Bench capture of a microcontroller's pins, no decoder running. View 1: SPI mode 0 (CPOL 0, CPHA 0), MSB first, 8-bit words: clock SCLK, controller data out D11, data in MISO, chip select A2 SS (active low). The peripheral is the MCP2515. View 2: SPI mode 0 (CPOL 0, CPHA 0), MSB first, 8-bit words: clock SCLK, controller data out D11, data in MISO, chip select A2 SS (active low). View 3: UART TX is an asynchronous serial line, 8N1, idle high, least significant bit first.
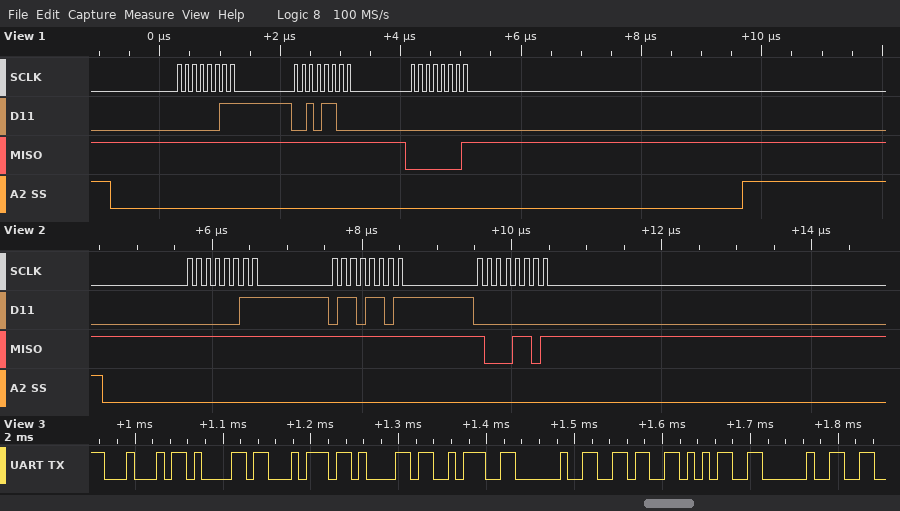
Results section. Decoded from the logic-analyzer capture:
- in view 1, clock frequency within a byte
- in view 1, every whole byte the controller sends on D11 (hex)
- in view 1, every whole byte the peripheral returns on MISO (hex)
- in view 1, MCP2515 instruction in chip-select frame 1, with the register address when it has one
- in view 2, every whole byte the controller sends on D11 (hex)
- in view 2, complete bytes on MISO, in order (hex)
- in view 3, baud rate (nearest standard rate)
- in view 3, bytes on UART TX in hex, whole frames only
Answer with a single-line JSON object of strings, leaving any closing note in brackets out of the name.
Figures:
{"in view 1, clock frequency within a byte": "8 MHz", "in view 1, every whole byte the controller sends on D11": "0x03 0x2C 0x00", "in view 1, every whole byte the peripheral returns on MISO": "0xFF 0xFF 0x01", "in view 1, MCP2515 instruction in chip-select frame 1, with the register address when it has one": "READ 0x2C", "in view 2, every whole byte the controller sends on D11": "03 6D 00", "in view 2, complete bytes on MISO, in order": "FF FF 8D", "in view 3, baud rate": "115200 baud", "in view 3, bytes on UART TX in hex, whole frames only": "44 61 74 61 3A 20 36 35 20"}
